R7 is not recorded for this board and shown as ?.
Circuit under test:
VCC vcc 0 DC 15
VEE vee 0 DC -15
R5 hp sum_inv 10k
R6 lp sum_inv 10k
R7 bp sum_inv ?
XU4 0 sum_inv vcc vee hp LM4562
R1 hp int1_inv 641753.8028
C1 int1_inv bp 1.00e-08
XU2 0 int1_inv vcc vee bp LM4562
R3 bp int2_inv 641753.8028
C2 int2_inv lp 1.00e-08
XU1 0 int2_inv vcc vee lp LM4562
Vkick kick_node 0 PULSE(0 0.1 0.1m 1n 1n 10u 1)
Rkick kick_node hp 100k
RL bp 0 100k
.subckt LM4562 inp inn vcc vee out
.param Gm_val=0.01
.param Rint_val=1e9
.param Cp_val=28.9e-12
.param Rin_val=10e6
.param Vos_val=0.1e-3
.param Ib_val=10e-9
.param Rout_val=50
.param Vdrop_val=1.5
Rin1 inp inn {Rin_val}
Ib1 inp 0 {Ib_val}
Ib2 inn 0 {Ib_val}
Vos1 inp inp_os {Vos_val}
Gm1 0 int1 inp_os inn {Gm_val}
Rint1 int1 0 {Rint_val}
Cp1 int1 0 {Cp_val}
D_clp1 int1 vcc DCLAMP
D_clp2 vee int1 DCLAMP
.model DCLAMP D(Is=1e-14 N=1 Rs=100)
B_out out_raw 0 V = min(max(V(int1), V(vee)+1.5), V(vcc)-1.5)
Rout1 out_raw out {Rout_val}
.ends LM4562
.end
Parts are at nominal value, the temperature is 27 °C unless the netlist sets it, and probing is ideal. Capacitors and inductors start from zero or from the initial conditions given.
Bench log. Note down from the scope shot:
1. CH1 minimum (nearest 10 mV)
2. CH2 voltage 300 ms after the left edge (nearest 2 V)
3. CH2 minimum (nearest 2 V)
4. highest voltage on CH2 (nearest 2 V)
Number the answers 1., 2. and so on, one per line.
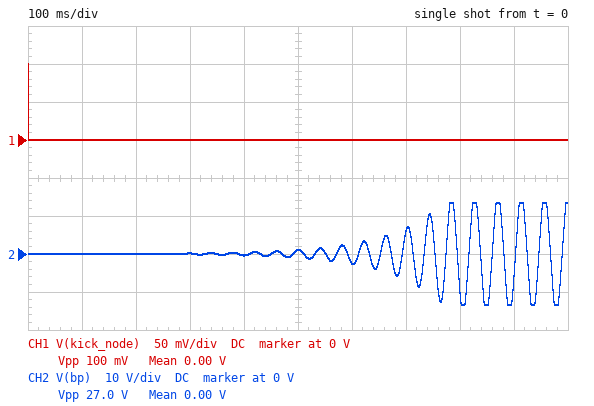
1. 0 V
2. 0 V
3. -14 V
4. 14 V
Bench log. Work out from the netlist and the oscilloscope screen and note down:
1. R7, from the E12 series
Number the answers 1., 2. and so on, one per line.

1. 82 kΩ
